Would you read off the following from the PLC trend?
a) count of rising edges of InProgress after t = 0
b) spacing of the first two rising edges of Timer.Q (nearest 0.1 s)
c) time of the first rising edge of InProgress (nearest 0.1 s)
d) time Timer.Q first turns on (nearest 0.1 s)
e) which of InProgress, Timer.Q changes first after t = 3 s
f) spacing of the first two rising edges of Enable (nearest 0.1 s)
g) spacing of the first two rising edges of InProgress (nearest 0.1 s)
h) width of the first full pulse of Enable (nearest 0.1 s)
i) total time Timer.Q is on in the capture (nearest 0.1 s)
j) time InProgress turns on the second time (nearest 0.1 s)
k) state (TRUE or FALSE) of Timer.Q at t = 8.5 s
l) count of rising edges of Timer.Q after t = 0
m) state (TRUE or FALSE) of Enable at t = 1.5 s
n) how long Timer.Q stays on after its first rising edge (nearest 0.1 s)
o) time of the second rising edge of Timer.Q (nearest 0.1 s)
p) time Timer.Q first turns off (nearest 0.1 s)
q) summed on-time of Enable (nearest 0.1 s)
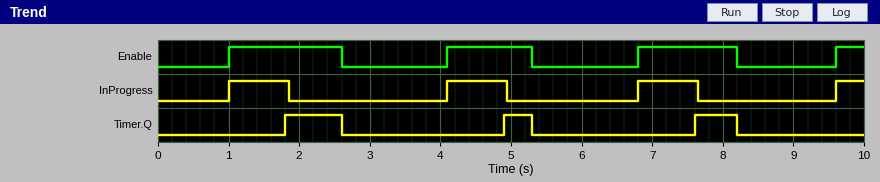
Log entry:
4
3.1 s
1.0 s
1.8 s
InProgress
3.1 s
3.1 s
1.6 s
1.8 s
4.1 s
FALSE
3
TRUE
0.8 s
4.9 s
2.6 s
4.6 s
